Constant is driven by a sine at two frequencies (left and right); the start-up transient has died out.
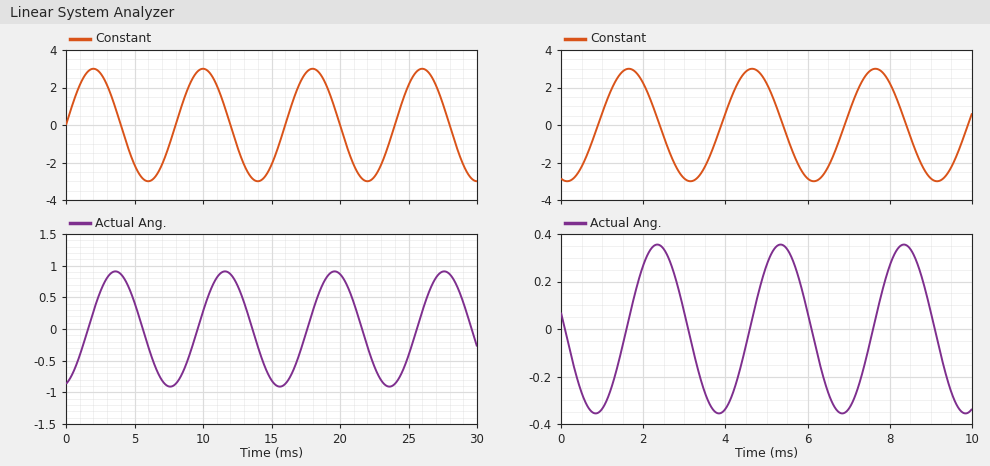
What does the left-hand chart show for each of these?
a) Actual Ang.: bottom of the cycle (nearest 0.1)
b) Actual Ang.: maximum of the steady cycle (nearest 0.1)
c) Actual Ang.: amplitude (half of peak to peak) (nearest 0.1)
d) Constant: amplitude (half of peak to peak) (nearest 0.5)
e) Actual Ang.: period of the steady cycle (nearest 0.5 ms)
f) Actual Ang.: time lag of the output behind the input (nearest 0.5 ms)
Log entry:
-0.9
0.9
0.9
3.0
8.0 ms
1.5 ms
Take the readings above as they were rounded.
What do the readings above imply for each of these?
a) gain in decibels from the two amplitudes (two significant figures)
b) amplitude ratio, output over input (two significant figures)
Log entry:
-10 dB
0.30
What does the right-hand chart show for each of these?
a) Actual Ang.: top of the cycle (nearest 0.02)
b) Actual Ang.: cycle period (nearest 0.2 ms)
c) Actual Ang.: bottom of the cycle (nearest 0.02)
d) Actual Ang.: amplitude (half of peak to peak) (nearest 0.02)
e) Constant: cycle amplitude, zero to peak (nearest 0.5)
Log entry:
0.36
3.0 ms
-0.36
0.36
3.0
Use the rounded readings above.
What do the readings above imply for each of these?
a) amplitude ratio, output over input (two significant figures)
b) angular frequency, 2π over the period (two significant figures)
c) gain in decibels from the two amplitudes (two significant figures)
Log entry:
0.12
2.1 rad/ms
-18 dB
